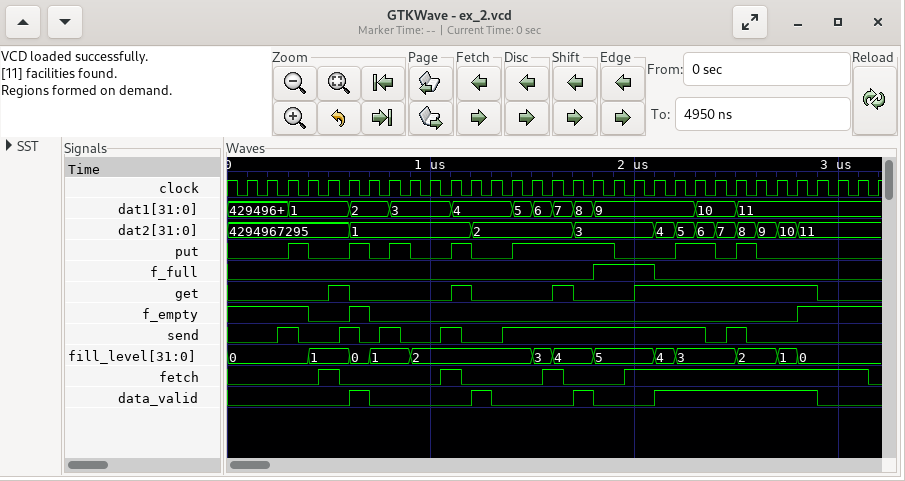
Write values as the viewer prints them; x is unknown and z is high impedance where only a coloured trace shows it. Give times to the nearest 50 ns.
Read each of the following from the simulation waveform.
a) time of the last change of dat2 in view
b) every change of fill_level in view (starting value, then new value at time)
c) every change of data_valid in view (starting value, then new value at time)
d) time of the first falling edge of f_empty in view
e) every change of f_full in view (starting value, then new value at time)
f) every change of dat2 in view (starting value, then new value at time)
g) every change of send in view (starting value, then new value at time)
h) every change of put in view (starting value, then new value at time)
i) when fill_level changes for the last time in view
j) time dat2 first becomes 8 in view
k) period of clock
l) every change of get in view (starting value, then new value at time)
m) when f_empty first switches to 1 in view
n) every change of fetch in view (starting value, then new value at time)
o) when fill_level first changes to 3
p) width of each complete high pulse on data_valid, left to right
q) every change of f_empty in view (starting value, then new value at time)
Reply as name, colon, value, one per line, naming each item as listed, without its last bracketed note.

time of the last change of dat2 in view: 2800 ns
every change of fill_level in view: 0, 1 at 400 ns, 0 at 600 ns, 1 at 700 ns, 2 at 900 ns, 3 at 1500 ns, 4 at 1600 ns, 5 at 1800 ns, 4 at 2100 ns, 3 at 2200 ns, 2 at 2500 ns, 1 at 2700 ns, 0 at 2800 ns
every change of data_valid in view: 0, 1 at 600 ns, 0 at 700 ns, 1 at 1200 ns, 0 at 1300 ns, 1 at 1700 ns, 0 at 1800 ns, 1 at 2100 ns, 0 at 2900 ns
time of the first falling edge of f_empty in view: 400 ns
every change of f_full in view: 0, 1 at 1800 ns, 0 at 2100 ns
every change of dat2 in view: 4294967295, 1 at 600 ns, 2 at 1200 ns, 3 at 1700 ns, 4 at 2100 ns, 5 at 2200 ns, 6 at 2300 ns, 7 at 2400 ns, 8 at 2500 ns, 9 at 2600 ns, 10 at 2700 ns, 11 at 2800 ns
every change of send in view: 0, 1 at 250 ns, 0 at 350 ns, 1 at 550 ns, 0 at 650 ns, 1 at 750 ns, 0 at 850 ns, 1 at 1050 ns, 0 at 1150 ns, 1 at 1350 ns, 0 at 2350 ns, 1 at 2450 ns, 0 at 2550 ns
every change of put in view: 0, 1 at 300 ns, 0 at 400 ns, 1 at 600 ns, 0 at 700 ns, 1 at 800 ns, 0 at 900 ns, 1 at 1100 ns, 0 at 1200 ns, 1 at 1400 ns, 0 at 1900 ns, 1 at 2200 ns, 0 at 2400 ns, 1 at 2500 ns, 0 at 2600 ns
when fill_level changes for the last time in view: 2800 ns
time dat2 first becomes 8 in view: 2500 ns
period of clock: 100 ns
every change of get in view: 0, 1 at 500 ns, 0 at 600 ns, 1 at 1100 ns, 0 at 1200 ns, 1 at 1600 ns, 0 at 1700 ns, 1 at 2000 ns, 0 at 2900 ns
when f_empty first switches to 1 in view: 600 ns
every change of fetch in view: 0, 1 at 450 ns, 0 at 550 ns, 1 at 1050 ns, 0 at 1150 ns, 1 at 1550 ns, 0 at 1650 ns, 1 at 1950 ns, 0 at 3150 ns
when fill_level first changes to 3: 1500 ns
width of each complete high pulse on data_valid, left to right: 100 ns, 100 ns, 100 ns, 800 ns
every change of f_empty in view: 1, 0 at 400 ns, 1 at 600 ns, 0 at 700 ns, 1 at 2800 ns
